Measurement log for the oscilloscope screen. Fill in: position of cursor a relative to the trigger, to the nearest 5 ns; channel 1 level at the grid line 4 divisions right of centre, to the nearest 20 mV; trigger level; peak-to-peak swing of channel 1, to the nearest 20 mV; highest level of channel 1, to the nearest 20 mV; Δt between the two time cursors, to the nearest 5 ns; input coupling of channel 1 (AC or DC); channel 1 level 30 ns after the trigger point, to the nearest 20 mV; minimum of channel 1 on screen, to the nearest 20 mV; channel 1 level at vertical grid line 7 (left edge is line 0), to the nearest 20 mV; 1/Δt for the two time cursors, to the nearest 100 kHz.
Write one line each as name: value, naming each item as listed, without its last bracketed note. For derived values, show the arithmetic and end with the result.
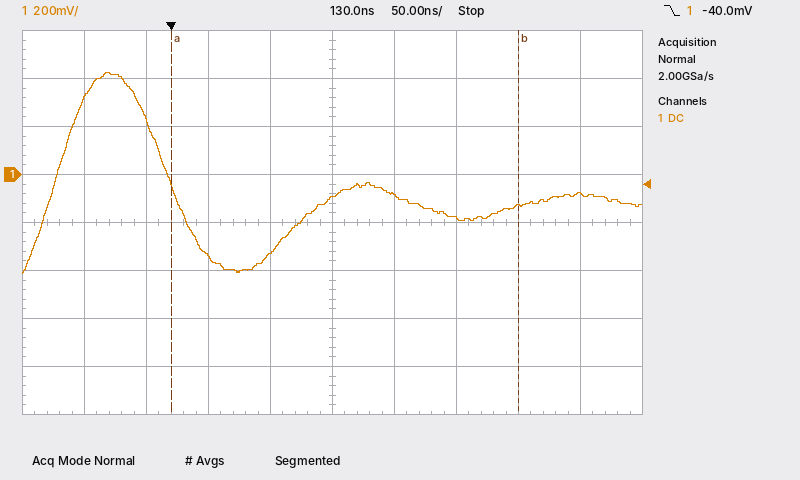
position of cursor a relative to the trigger, to the nearest 5 ns: 0 ns
channel 1 level at the grid line 4 divisions right of centre, to the nearest 20 mV: -80 mV
trigger level: -40.0 mV
peak-to-peak swing of channel 1, to the nearest 20 mV: 420 mV − (-420 mV) = 840 mV
highest level of channel 1, to the nearest 20 mV: 420 mV
Δt between the two time cursors, to the nearest 5 ns: 280 ns
input coupling of channel 1: DC
channel 1 level 30 ns after the trigger point, to the nearest 20 mV: -340 mV
minimum of channel 1 on screen, to the nearest 20 mV: -420 mV
channel 1 level at vertical grid line 7 (left edge is line 0), to the nearest 20 mV: -180 mV
1/Δt for the two time cursors, to the nearest 100 kHz: 1 / 280 ns ≈ 3.6 MHz
